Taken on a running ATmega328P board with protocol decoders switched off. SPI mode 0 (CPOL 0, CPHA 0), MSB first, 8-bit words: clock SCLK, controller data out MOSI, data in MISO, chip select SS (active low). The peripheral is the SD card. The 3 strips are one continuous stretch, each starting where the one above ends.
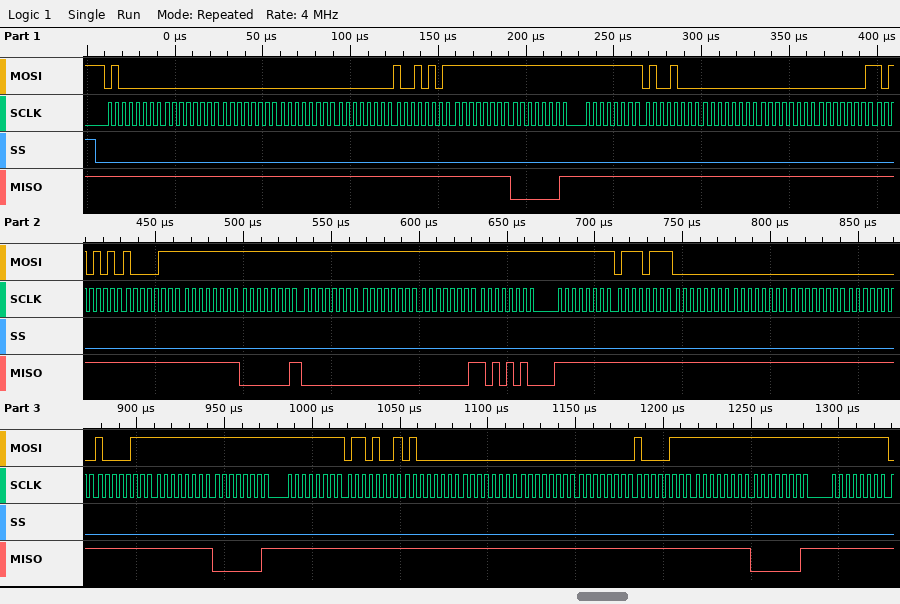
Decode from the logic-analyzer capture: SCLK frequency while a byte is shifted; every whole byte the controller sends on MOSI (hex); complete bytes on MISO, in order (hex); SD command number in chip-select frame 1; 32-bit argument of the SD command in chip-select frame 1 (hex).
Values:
250 kHz
40 00 00 00 00 95 FF FF FF 48 00 00 01 AA 87 FF FF FF FF FF FF FF 77 00 00 00 00 87 FF FF FF 69 40 00 00 00 87 FF FF FF
FF FF FF FF FF FF FF 01 FF FF FF FF FF FF FF FF 01 00 00 01 AA FF FF FF FF FF FF FF FF 01 FF FF FF FF FF FF FF FF 01 FF
CMD0
0x00000000
